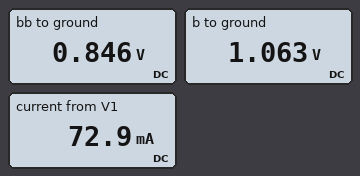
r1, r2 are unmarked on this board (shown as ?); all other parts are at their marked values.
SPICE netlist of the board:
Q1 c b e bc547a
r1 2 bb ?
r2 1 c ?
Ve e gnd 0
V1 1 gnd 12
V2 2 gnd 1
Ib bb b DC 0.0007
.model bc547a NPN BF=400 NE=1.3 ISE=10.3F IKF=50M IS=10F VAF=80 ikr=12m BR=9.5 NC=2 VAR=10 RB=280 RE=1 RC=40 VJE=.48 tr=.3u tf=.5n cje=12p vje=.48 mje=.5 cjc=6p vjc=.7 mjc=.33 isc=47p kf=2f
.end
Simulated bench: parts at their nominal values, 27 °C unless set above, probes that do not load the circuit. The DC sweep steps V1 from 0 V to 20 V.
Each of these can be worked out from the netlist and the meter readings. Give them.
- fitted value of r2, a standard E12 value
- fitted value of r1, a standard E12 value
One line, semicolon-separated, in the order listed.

120 Ω; 220 Ω
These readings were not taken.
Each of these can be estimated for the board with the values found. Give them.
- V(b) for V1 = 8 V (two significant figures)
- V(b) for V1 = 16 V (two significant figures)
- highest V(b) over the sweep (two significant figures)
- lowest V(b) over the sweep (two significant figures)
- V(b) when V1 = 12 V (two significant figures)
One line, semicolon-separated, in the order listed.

1.0 V; 1.1 V; 1.1 V; 900 mV; 1.1 V
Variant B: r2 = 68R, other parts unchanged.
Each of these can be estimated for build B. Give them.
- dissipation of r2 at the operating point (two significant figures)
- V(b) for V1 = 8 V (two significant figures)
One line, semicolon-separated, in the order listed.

400 mW; 1.1 V
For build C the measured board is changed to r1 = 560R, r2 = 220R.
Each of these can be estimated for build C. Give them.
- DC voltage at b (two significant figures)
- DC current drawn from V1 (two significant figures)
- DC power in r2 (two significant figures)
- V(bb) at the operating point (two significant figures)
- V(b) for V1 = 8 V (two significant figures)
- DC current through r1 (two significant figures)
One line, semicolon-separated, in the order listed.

1.0 V; 46 mA; 460 mW; 610 mV; 990 mV; 700 µA
